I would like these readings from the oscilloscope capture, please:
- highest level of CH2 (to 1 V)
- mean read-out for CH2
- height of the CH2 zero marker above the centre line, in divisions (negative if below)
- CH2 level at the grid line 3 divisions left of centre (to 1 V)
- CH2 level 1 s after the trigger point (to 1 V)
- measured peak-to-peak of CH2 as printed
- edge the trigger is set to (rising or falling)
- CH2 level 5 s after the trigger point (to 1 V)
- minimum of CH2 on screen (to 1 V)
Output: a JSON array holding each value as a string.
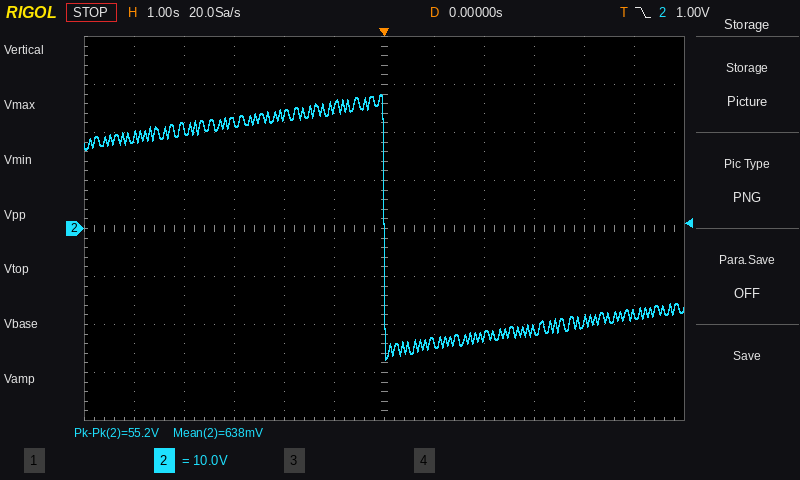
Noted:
["28 V", "638 mV", "0.0 div", "22 V", "-24 V", "55.2 V", "falling", "-18 V", "-27 V"]
